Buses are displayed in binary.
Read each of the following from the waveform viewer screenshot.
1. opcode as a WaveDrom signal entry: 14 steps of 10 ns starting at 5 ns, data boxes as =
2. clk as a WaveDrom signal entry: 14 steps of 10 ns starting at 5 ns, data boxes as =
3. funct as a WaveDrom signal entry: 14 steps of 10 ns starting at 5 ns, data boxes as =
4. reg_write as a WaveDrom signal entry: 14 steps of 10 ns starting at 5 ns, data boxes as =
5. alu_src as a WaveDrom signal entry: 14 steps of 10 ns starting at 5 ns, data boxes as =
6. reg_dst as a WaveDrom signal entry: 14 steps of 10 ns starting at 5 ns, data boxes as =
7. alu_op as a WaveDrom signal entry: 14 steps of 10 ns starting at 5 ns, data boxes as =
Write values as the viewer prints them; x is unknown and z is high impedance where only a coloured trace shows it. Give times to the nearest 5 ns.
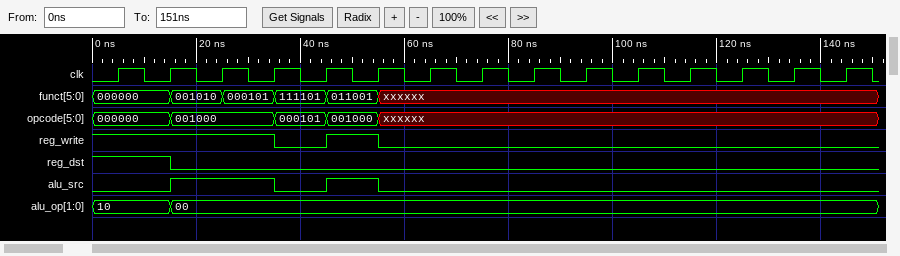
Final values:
{name: 'opcode', wave: '==.==x........', data: '000000 001000 000101 001000'}
{name: 'clk', wave: 'p.............'}
{name: 'funct', wave: '=====x........', data: '000000 001010 000101 111101 011001'}
{name: 'reg_write', wave: '1..010........'}
{name: 'alu_src', wave: '01.010........'}
{name: 'reg_dst', wave: '10............'}
{name: 'alu_op', wave: '==............', data: '10 00'}
